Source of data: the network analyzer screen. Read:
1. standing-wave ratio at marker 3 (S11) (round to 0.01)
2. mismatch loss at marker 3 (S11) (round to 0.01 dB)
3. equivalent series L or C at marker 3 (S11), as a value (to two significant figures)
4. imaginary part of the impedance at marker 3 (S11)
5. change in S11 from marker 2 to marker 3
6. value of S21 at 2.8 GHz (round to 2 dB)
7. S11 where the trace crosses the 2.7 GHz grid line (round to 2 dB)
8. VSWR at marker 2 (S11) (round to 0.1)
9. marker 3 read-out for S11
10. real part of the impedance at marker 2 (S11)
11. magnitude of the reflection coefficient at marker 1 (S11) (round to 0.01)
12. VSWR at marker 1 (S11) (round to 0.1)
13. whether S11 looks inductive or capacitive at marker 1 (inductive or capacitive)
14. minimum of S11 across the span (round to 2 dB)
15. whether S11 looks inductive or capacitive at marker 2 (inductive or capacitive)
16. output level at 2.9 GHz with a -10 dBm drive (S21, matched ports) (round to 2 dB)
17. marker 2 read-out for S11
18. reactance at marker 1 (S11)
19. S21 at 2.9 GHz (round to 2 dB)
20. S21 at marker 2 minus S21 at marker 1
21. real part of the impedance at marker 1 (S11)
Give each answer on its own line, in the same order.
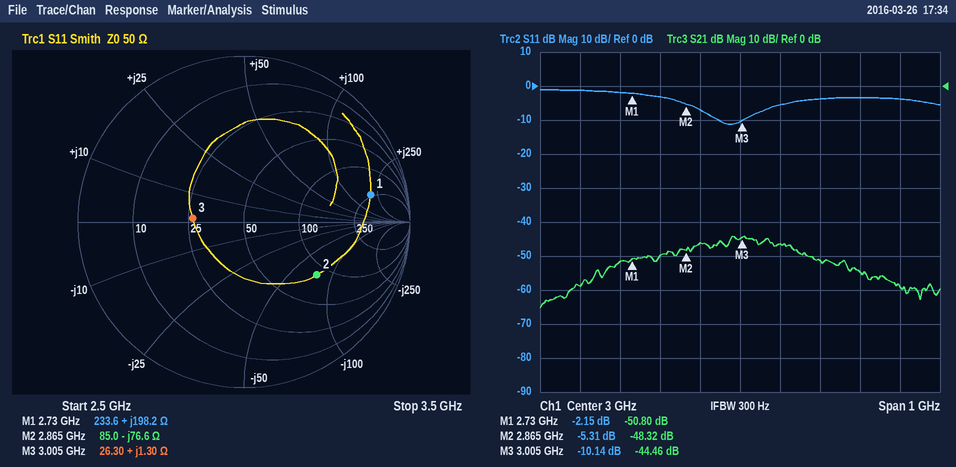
1.90
0.44 dB
69 pH
+1.30 Ω
-4.83 dB
-50 dB
-2 dB
3.4
-10.14 dB
85.0 Ω
0.78
8.1
inductive
-12 dB
capacitive
-56 dBm
-5.31 dB
+198.2 Ω
-46 dB
2.48 dB
233.6 Ω
